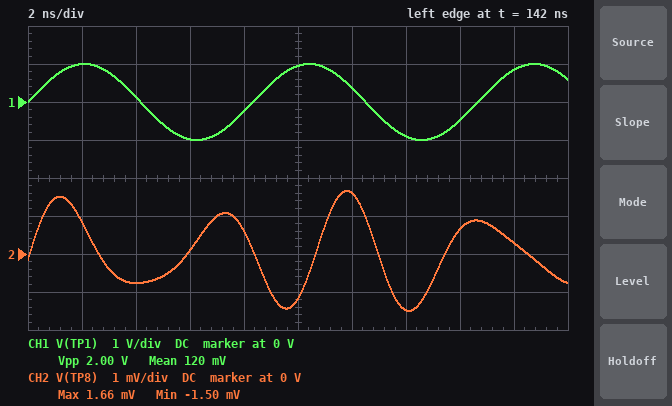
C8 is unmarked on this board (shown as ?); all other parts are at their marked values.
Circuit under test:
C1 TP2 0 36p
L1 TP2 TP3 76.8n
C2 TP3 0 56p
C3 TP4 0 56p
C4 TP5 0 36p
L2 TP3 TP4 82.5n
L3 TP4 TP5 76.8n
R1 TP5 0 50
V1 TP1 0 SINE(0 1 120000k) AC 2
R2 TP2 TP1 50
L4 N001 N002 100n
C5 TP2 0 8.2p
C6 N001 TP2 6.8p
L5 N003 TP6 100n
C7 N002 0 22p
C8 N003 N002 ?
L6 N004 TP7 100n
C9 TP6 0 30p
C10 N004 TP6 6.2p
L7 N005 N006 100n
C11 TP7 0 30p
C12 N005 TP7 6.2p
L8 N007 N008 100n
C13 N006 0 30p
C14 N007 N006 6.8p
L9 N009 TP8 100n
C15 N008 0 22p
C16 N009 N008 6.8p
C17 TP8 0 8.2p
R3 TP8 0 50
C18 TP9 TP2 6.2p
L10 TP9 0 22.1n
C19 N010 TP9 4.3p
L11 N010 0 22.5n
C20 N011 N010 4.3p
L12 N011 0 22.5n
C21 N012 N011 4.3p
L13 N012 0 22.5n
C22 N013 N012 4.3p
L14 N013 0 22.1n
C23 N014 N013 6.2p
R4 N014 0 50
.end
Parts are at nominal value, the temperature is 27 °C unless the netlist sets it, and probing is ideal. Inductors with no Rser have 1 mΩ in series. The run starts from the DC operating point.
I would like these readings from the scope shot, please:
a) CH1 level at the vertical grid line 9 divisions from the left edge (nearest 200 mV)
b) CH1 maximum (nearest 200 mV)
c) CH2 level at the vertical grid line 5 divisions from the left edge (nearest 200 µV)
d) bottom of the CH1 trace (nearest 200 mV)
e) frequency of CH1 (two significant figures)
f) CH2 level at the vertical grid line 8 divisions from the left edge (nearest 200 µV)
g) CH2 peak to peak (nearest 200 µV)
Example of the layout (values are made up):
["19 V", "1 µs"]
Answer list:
["800 mV", "1.0 V", "-1.2 mV", "-1.0 V", "120 MHz", "600 µV", "3.2 mV"]
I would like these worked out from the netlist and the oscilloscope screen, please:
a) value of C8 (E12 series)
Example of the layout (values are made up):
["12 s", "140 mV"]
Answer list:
["8.2 pF"]
